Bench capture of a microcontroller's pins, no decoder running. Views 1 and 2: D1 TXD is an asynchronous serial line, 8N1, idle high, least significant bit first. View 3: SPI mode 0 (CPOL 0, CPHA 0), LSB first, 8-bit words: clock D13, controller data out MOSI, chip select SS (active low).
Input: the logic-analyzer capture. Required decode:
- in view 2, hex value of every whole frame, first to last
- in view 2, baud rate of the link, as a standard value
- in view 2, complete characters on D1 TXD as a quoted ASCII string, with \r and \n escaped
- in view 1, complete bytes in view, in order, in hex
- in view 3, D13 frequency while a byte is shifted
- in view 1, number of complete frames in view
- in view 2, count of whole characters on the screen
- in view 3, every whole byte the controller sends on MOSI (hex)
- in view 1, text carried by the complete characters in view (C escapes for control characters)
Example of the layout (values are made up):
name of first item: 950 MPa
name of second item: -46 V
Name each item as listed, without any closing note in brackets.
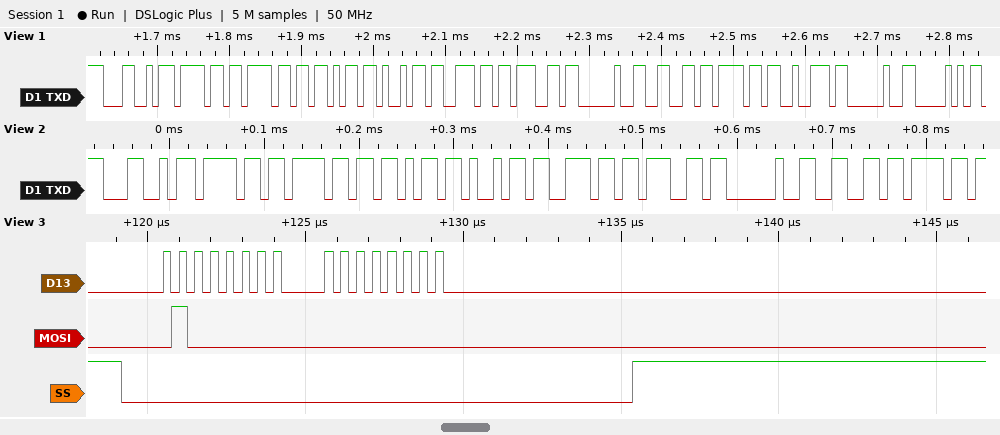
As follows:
in view 2, hex value of every whole frame, first to last: 4C 6F 6F 6B 69 6E 67 20 66 6F
in view 2, baud rate of the link, as a standard value: 115200 baud
in view 2, complete characters on D1 TXD as a quoted ASCII string, with \r and \n escaped: "Looking fo"
in view 1, complete bytes in view, in order, in hex: 0x4C 0x6F 0x6F 0x6B 0x69 0x6E 0x67 0x20 0x66 0x6F 0x72 0x20 0x50
in view 3, D13 frequency while a byte is shifted: 2 MHz
in view 1, number of complete frames in view: 13
in view 2, count of whole characters on the screen: 10
in view 3, every whole byte the controller sends on MOSI: 0x02 0x00
in view 1, text carried by the complete characters in view: "Looking for P"
